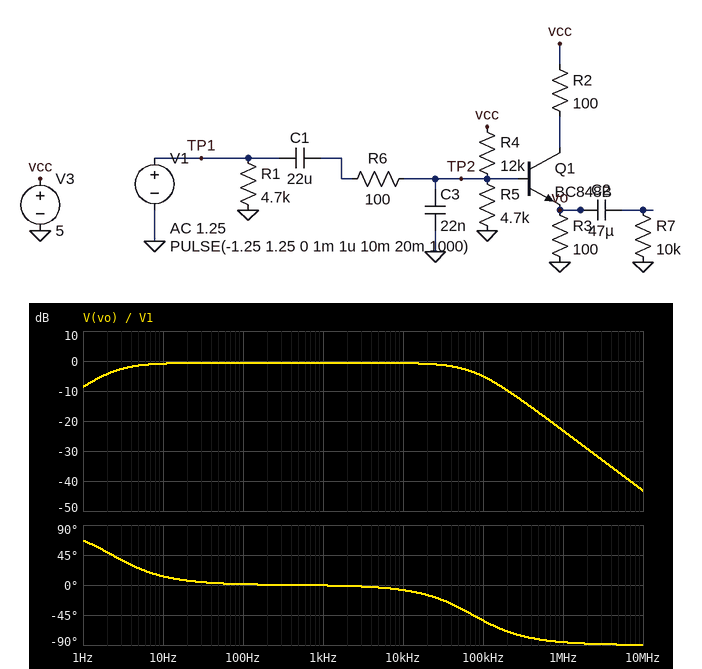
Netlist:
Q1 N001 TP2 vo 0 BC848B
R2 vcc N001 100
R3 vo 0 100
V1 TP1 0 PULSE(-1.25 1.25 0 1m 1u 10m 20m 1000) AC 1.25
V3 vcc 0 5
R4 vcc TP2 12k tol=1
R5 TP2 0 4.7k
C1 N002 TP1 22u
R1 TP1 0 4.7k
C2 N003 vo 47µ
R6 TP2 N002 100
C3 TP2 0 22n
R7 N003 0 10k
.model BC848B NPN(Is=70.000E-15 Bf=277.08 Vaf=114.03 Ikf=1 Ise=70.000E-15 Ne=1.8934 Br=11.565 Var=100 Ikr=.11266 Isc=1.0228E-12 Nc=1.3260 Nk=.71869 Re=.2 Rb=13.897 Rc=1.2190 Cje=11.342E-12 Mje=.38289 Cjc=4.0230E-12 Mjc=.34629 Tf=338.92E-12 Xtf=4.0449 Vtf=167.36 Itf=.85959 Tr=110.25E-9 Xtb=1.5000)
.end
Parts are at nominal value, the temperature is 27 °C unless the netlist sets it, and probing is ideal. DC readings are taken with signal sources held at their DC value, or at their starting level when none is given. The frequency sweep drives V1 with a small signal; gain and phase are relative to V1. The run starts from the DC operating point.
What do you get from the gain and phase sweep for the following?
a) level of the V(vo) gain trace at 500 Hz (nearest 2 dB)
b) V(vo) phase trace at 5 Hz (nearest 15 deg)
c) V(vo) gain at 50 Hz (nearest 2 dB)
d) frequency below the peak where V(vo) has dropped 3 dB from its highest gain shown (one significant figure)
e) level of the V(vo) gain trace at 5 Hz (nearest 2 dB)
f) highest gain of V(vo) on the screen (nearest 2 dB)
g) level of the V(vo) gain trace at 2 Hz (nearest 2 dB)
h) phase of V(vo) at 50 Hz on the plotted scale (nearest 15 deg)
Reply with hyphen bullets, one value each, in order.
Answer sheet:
- 0 dB
- 30 deg
- 0 dB
- 2 Hz
- -2 dB
- 0 dB
- -4 dB
- 0 deg
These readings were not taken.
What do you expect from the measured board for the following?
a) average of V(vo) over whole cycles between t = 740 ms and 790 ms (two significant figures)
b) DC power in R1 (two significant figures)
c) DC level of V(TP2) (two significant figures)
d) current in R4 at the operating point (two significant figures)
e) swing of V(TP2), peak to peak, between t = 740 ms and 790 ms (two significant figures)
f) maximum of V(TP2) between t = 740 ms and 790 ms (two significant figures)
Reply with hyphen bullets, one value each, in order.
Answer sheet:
- 920 mV
- 330 µW
- 1.3 V
- 310 µA
- 2.6 V
- 2.5 V
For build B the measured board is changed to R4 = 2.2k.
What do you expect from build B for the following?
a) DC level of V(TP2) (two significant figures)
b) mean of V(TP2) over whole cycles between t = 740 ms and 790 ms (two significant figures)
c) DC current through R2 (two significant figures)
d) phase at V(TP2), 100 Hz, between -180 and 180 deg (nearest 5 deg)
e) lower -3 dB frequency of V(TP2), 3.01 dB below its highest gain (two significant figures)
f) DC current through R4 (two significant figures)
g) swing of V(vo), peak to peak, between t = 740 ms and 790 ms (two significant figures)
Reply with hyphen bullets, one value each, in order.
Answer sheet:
- 3.1 V
- 2.3 V
- 24 mA
- 15 deg
- 24 Hz
- 850 µA
- 2.4 V
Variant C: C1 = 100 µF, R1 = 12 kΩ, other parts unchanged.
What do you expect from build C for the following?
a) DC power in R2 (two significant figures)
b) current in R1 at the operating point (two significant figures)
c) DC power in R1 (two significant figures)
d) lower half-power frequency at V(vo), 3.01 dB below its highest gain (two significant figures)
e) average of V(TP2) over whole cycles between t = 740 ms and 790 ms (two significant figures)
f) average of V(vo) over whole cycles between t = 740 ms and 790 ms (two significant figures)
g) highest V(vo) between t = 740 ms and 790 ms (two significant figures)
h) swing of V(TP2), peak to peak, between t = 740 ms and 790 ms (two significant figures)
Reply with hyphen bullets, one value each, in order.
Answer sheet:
- 4.5 mW
- 100 µA
- 130 µW
- 510 mHz
- 1.4 V
- 960 mV
- 1.9 V
- 2.5 V
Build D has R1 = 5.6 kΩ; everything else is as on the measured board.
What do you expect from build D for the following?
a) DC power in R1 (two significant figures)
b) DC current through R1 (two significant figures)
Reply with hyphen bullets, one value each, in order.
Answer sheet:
- 280 µW
- 220 µA
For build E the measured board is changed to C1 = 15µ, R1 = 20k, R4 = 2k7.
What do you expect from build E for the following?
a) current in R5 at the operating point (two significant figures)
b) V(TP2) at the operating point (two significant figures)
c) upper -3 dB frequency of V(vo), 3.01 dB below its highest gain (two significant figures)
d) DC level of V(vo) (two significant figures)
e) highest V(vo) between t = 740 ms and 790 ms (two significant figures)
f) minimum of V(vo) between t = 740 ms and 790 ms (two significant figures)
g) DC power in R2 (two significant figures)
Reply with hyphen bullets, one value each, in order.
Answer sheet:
- 640 µA
- 3.0 V
- 77 kHz
- 2.3 V
- 2.7 V
- 170 mV
- 54 mW
